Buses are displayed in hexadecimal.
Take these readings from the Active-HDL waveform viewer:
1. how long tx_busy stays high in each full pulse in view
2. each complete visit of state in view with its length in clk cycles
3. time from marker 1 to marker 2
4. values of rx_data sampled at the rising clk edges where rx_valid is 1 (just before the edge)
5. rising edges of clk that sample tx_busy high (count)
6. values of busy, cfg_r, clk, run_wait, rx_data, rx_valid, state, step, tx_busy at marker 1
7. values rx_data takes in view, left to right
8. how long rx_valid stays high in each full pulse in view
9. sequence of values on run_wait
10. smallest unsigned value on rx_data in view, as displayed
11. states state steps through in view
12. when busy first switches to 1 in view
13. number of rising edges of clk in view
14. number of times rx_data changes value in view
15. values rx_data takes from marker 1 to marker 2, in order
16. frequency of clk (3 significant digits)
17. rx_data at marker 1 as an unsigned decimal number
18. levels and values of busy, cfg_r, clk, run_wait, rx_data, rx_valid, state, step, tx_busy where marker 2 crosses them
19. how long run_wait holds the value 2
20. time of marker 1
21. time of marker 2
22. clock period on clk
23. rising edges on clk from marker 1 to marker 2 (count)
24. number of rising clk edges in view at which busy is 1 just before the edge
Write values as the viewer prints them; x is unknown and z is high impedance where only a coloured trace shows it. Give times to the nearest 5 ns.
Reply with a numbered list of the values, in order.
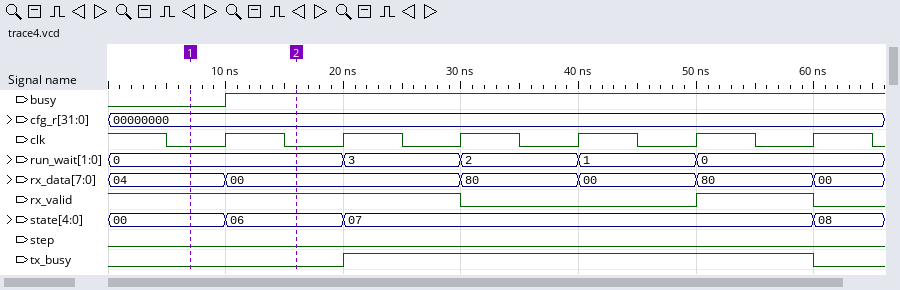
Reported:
1. 40 ns
2. 06: 1, 07: 4
3. 10 ns
4. 04, 00, 00, 80
5. 4
6. busy=0, cfg_r=00000000, clk=0, run_wait=0, rx_data=04, rx_valid=1, state=00, step=0, tx_busy=0
7. 04, 00, 80, 00, 80, 00
8. 10 ns
9. 0, 3, 2, 1, 0
10. 00
11. 00, 06, 07, 08
12. 10 ns
13. 6
14. 5
15. 04, 00
16. 100 MHz
17. 4
18. busy=1, cfg_r=00000000, clk=0, run_wait=0, rx_data=00, rx_valid=1, state=06, step=0, tx_busy=0
19. 10 ns
20. 5 ns
21. 15 ns
22. 10 ns
23. 1
24. 5
